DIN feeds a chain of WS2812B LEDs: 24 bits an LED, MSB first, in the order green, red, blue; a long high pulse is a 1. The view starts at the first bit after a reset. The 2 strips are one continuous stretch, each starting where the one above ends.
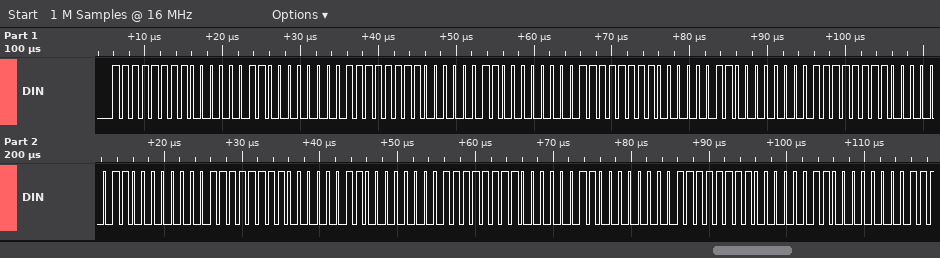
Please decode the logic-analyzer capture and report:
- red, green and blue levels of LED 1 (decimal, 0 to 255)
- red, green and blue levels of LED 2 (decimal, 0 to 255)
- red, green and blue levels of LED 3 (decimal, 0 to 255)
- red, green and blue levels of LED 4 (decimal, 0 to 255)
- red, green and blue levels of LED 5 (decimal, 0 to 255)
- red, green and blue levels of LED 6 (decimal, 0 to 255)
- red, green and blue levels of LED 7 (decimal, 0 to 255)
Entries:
3, 255, 0
3, 255, 0
3, 255, 0
3, 255, 0
3, 255, 0
3, 255, 0
3, 255, 0
